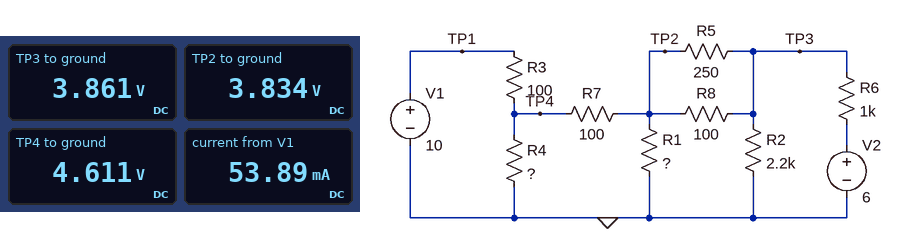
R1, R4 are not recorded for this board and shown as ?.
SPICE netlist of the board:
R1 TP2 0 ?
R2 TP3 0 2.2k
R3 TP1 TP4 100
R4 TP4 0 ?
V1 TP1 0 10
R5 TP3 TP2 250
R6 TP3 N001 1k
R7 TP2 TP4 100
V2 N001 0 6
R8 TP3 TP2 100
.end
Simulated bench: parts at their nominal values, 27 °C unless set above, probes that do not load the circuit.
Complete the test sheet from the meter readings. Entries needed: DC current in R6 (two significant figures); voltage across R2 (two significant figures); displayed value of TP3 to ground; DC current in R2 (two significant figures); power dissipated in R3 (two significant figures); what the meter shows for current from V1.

2.1 mA
3.9 V
3.861 V
1.8 mA
290 mW
53.89 mA
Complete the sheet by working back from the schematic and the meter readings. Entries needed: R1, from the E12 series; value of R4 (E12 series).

470 Ω
100 Ω
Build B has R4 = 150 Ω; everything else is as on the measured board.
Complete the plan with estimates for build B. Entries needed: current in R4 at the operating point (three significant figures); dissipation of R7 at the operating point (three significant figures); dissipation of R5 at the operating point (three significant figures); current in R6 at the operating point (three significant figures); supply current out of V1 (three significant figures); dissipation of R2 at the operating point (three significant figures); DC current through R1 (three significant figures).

36.1 mA
9.65 mW
3.26 µW
1.60 mA
45.9 mA
8.80 mW
9.42 mA
